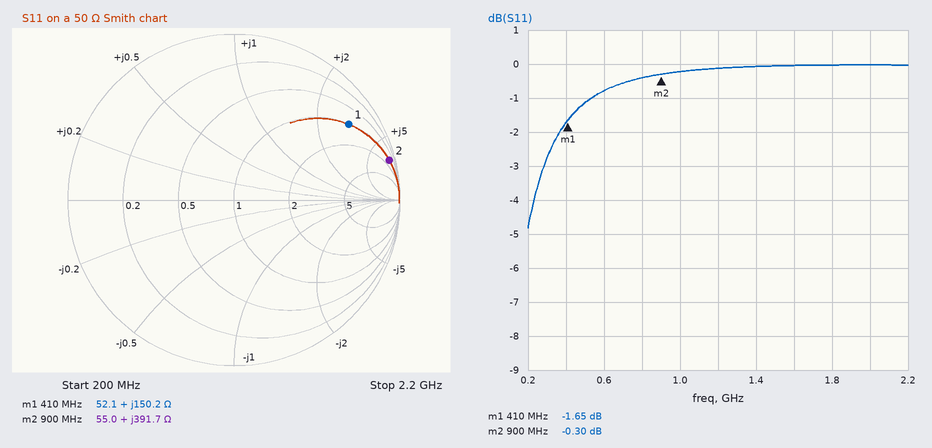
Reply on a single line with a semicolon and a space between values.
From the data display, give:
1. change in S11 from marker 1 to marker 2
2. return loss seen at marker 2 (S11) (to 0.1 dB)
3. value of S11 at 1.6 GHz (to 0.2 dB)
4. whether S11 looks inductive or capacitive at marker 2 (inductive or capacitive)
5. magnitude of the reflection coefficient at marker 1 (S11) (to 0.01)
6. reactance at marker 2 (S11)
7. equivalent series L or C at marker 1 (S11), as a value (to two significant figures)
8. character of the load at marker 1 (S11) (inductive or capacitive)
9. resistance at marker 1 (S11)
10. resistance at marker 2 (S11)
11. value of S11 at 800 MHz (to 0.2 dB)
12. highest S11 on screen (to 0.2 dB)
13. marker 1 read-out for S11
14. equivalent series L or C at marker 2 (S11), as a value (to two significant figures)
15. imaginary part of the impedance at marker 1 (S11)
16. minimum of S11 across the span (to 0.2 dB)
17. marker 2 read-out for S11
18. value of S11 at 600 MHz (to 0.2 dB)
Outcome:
1.35 dB; 0.3 dB; 0.0 dB; inductive; 0.83; +391.7 Ω; 58 nH; inductive; 52.1 Ω; 55.0 Ω; -0.4 dB; 0.0 dB; -1.65 dB; 69 nH; +150.2 Ω; -4.8 dB; -0.30 dB; -0.8 dB
